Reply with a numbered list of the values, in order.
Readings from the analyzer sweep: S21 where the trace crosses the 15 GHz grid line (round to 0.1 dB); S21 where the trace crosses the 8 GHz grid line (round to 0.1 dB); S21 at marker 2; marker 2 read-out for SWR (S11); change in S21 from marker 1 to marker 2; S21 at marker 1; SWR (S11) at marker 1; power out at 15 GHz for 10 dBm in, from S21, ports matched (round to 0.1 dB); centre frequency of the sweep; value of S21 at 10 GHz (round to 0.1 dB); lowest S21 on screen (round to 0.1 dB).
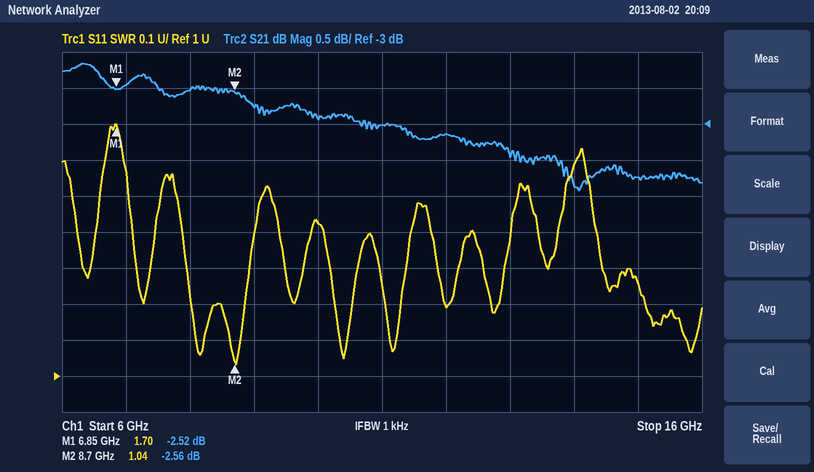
1. -3.7 dB
2. -2.5 dB
3. -2.56 dB
4. 1.04
5. -0.04 dB
6. -2.52 dB
7. 1.70
8. 6.3 dBm
9. 11 GHz
10. -2.9 dB
11. -3.9 dB
